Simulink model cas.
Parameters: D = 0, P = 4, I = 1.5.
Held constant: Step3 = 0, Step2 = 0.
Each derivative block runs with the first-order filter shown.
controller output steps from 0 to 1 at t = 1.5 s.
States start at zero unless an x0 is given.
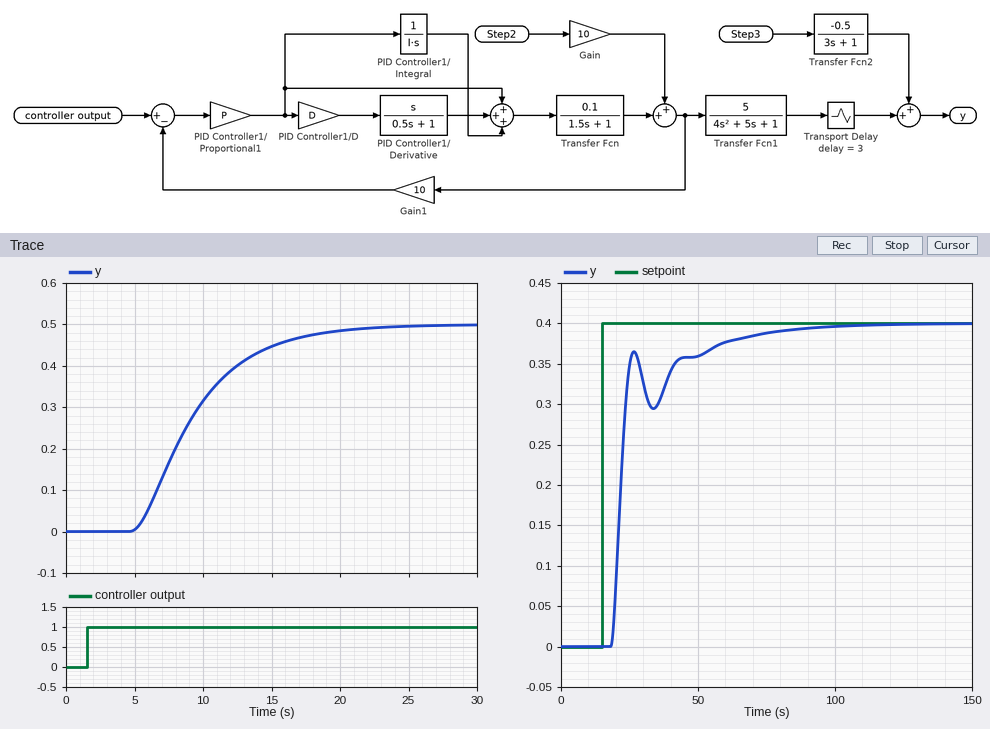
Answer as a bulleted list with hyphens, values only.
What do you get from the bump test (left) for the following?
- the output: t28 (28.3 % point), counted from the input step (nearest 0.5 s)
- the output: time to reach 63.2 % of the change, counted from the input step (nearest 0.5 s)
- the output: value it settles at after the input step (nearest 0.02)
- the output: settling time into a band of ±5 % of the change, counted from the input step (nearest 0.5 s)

- 5.5 s
- 8.5 s
- 0.50
- 16.5 s
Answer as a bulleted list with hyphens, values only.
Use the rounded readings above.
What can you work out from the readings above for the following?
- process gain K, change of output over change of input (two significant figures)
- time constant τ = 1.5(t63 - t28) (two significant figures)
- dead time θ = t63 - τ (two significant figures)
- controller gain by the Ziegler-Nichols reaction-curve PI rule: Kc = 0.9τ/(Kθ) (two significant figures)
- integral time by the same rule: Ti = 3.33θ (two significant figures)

- 0.50
- 4.5 s
- 4.0 s
- 2.0
- 13 s
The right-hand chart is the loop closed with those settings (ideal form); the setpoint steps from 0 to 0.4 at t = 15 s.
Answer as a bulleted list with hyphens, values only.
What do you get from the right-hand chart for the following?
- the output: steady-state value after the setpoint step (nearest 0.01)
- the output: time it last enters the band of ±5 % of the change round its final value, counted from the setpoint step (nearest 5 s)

- 0.40
- 50 s
